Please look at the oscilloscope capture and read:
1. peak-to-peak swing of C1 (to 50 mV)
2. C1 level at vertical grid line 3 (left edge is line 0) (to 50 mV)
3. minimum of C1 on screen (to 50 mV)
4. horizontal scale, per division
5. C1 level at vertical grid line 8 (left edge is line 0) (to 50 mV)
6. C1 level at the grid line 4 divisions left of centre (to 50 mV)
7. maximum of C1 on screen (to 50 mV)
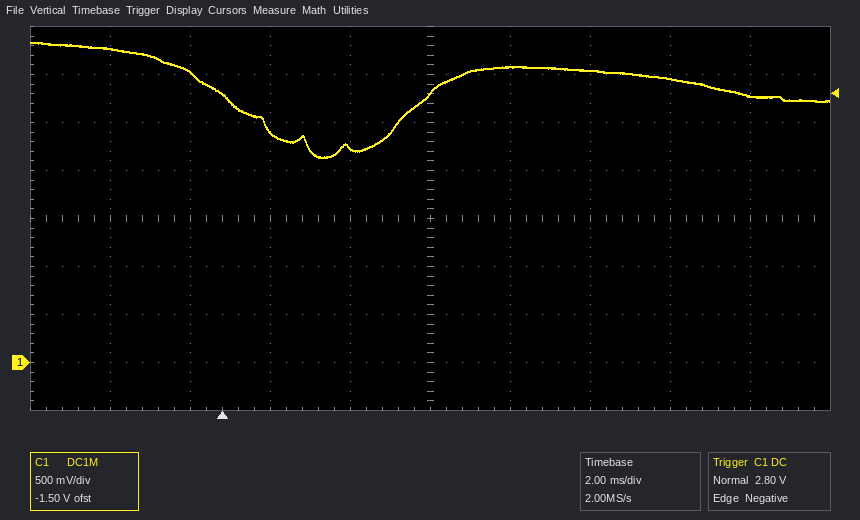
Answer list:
1.20 V
2.40 V
2.15 V
2 ms
2.95 V
3.25 V
3.35 V
